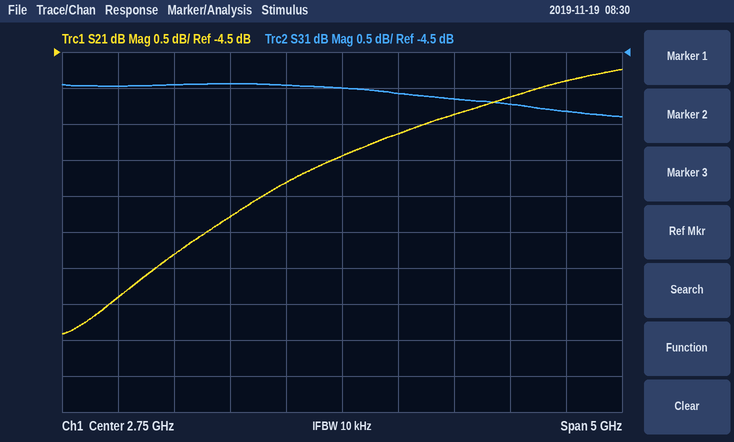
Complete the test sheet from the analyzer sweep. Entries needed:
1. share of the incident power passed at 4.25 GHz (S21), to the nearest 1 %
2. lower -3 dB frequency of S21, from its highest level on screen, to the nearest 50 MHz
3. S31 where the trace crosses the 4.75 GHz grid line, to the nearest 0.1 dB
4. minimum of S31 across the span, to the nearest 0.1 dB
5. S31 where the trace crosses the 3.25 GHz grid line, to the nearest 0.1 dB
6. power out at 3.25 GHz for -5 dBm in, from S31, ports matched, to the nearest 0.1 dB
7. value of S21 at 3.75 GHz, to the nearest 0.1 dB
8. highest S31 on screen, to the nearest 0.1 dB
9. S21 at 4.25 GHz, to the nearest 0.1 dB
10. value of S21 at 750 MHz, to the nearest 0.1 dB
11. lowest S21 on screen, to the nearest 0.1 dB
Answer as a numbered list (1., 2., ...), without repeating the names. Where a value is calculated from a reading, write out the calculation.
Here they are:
1. 10^(-5.1/10) ≈ 31 %
2. 900 MHz
3. -5.3 dB
4. -5.4 dB
5. -5.1 dB
6. -5 dBm + (-5.1 dB) = -10.1 dBm
7. -5.4 dB
8. -4.9 dB
9. -5.1 dB
10. -7.9 dB
11. -8.4 dB
